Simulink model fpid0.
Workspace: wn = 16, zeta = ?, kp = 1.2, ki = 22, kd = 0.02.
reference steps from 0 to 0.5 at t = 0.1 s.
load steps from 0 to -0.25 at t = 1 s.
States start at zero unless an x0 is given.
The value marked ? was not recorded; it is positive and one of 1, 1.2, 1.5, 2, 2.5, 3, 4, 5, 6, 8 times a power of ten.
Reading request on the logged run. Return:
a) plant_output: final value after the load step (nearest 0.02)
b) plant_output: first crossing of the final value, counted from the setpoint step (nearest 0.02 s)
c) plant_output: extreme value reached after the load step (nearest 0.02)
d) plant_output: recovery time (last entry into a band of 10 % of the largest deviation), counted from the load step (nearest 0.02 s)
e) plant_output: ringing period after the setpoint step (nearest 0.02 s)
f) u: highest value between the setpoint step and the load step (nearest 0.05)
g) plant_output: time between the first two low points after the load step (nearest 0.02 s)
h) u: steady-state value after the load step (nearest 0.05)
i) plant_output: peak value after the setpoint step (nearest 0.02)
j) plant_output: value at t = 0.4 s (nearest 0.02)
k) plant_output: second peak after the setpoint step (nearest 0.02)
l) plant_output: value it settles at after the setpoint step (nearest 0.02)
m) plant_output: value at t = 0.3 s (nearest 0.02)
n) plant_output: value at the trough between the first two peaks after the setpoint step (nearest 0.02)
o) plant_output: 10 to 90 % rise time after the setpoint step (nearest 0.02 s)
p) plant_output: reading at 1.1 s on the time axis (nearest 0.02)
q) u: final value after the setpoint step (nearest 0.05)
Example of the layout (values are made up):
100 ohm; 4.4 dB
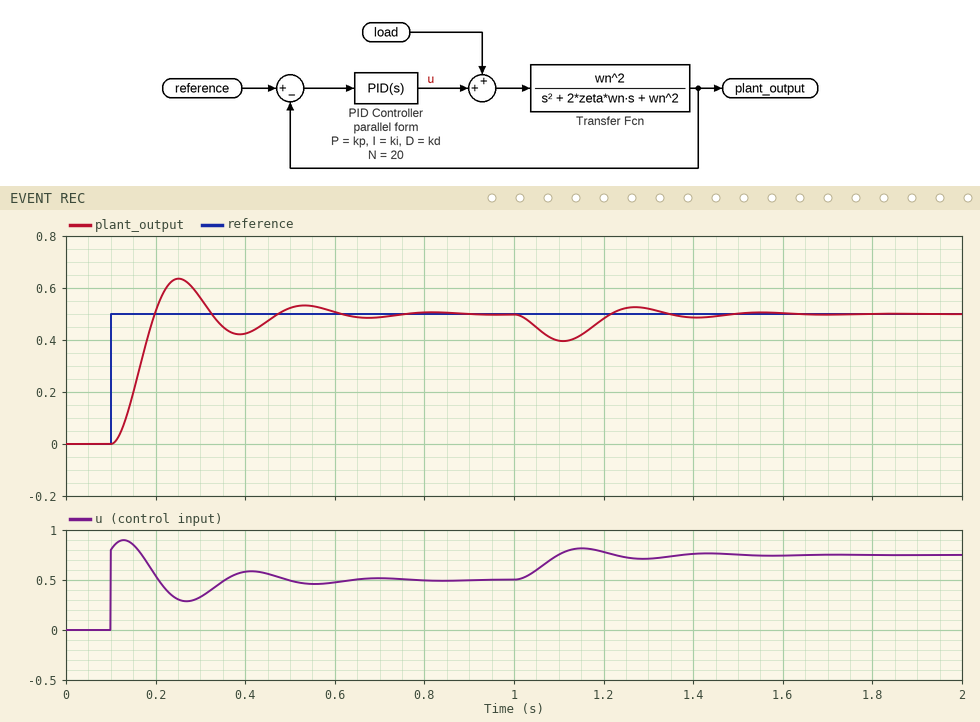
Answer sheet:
0.50; 0.10 s; 0.40; 0.44 s; 0.28 s; 0.90; 0.30 s; 0.75; 0.64; 0.42; 0.54; 0.50; 0.56; 0.42; 0.06 s; 0.40; 0.50
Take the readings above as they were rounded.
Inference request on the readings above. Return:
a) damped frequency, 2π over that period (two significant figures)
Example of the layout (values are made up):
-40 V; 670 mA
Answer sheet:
22 rad/s
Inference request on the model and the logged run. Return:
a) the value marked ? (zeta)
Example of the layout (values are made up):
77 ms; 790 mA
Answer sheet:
0.6
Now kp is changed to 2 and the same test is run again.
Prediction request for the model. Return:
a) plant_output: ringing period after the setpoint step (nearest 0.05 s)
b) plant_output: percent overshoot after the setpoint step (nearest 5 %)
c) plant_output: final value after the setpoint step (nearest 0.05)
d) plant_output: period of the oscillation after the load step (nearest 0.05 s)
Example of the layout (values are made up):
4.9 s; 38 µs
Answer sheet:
0.25 s; 25 %; 0.50; 0.25 s
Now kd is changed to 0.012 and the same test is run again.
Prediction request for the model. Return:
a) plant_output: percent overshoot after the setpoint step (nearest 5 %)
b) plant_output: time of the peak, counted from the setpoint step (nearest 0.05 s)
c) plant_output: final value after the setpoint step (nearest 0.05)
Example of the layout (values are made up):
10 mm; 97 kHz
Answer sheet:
30 %; 0.15 s; 0.50
